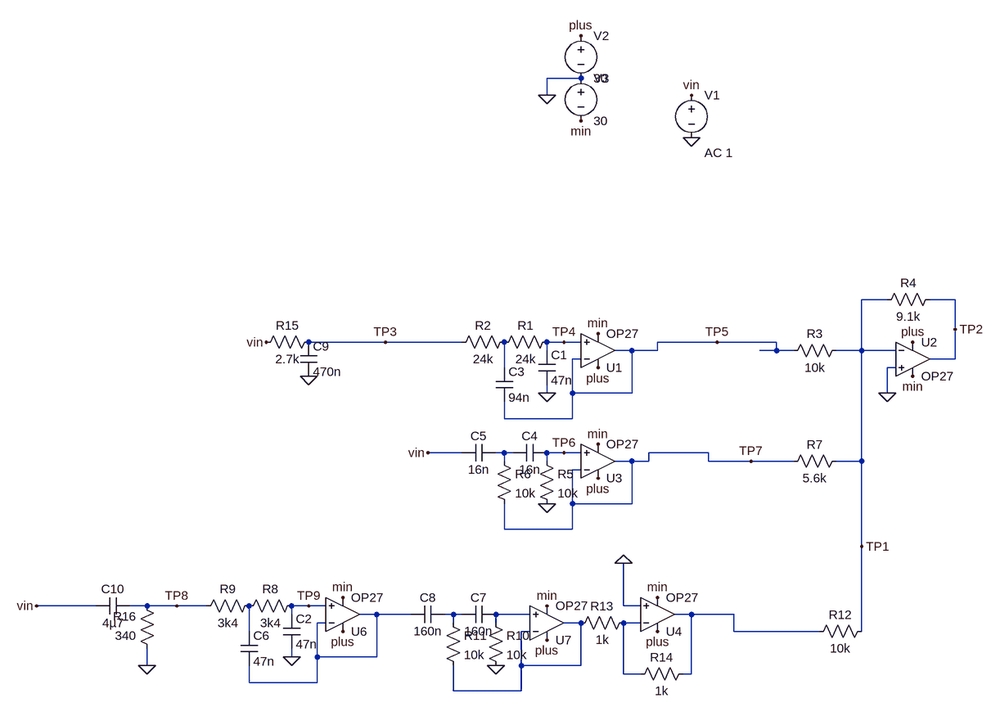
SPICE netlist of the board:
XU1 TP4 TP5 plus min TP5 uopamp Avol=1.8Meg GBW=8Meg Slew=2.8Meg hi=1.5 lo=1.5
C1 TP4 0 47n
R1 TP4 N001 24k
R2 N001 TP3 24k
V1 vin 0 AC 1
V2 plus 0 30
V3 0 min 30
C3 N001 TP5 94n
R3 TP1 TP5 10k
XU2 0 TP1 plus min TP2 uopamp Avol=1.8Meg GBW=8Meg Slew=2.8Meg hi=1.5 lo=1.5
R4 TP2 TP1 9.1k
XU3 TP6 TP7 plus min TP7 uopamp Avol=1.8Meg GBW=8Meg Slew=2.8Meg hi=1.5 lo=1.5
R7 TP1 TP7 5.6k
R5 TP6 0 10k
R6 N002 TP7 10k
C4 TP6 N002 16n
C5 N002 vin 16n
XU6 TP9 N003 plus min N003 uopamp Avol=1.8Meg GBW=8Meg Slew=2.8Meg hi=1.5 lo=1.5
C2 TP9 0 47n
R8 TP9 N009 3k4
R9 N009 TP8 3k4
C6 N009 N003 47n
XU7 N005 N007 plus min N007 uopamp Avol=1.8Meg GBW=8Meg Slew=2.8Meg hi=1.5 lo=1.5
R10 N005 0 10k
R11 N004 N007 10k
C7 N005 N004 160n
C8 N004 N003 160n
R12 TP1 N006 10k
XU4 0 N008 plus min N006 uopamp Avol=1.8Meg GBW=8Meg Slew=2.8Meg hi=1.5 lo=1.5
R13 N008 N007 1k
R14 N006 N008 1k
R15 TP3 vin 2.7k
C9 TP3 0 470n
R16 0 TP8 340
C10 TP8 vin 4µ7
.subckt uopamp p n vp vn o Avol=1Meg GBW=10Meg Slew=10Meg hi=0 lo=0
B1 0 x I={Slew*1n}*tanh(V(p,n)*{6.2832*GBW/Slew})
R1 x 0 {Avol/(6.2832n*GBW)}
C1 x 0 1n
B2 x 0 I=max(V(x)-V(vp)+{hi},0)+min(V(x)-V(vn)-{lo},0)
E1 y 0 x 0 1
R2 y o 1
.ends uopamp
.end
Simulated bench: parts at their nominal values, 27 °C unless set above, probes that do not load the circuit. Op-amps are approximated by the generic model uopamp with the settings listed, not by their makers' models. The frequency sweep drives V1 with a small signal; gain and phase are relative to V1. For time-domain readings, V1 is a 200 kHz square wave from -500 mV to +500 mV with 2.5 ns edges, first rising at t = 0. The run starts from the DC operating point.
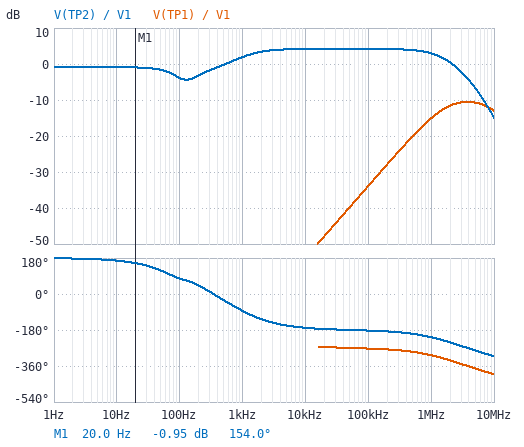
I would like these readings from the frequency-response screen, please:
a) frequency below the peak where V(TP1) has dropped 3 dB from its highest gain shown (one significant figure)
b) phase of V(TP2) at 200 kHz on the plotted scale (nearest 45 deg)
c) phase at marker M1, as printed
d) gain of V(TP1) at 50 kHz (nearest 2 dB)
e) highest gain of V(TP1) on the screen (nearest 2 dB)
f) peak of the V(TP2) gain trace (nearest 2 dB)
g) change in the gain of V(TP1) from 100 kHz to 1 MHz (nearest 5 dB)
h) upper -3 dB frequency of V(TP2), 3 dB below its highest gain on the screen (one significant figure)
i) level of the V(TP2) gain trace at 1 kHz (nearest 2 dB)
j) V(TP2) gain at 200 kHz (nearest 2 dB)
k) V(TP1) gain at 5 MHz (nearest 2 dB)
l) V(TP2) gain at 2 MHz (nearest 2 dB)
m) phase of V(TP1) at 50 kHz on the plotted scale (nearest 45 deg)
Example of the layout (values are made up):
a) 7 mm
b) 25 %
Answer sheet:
a) 1 MHz
b) -180 deg
c) 154.0 deg
d) -40 dB
e) -10 dB
f) 4 dB
g) 20 dB
h) 2 MHz
i) 2 dB
j) 4 dB
k) -10 dB
l) 0 dB
m) -270 deg
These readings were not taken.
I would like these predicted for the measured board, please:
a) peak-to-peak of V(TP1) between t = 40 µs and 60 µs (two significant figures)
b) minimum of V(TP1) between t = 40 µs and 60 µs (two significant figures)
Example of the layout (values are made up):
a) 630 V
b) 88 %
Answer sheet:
a) 330 mV
b) -170 mV
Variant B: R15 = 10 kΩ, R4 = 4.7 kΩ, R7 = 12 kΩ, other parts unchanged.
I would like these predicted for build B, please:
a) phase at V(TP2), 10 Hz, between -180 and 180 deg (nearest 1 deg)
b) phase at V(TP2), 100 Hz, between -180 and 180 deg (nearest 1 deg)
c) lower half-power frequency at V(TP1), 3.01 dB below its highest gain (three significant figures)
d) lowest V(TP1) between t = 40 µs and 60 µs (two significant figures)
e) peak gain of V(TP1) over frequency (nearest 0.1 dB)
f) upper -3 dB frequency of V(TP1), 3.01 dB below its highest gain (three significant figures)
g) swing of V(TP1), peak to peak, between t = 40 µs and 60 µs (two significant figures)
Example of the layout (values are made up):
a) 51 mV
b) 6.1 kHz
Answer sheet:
a) 154 deg
b) 89 deg
c) 2.04 MHz
d) -23 mV
e) -18.6 dB
f) 13.5 MHz
g) 46 mV
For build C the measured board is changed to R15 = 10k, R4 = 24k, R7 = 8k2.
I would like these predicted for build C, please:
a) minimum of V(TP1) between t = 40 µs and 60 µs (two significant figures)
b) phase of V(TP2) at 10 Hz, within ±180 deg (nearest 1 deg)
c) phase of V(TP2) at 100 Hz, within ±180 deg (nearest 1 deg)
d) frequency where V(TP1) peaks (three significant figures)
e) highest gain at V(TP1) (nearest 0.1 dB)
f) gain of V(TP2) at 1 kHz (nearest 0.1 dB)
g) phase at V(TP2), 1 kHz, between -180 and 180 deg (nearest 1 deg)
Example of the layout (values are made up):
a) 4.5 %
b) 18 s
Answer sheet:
a) -230 mV
b) 154 deg
c) 88 deg
d) 2.71 MHz
e) -10.4 dB
f) 8.3 dB
g) -83 deg
